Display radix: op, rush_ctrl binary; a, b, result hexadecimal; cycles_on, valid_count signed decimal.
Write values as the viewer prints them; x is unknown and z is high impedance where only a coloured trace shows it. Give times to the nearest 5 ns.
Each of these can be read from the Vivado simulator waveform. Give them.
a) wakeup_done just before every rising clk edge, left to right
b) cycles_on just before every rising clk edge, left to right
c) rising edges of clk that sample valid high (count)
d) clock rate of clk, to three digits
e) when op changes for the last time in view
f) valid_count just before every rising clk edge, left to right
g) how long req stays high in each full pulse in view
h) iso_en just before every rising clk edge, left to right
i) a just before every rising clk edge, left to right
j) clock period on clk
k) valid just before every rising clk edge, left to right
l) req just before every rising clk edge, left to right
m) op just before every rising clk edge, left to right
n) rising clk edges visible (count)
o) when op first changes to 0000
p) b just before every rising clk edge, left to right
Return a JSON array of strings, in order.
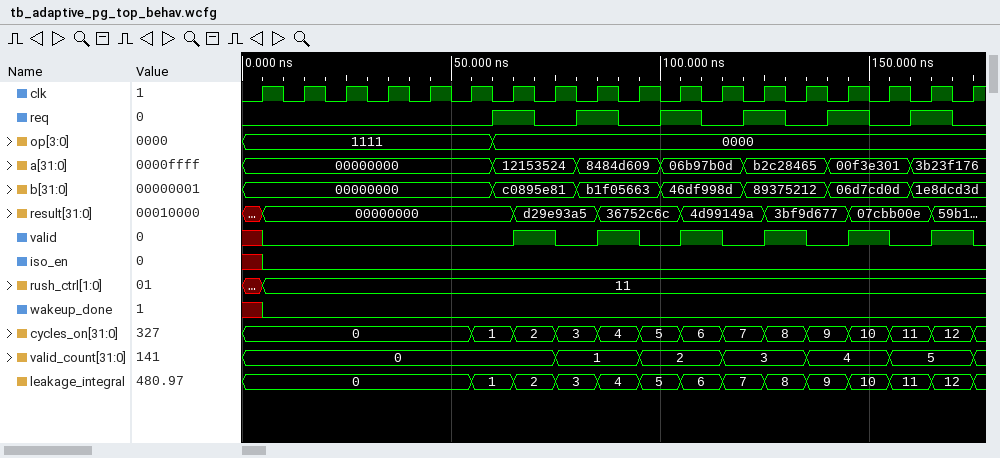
["x 0 0 0 0 0 0 0 0 0 0 0 0 0 0 0 0 0", "0, 0, 0, 0, 0, 0, 1, 2, 3, 4, 5, 6, 7, 8, 9, 10, 11, 12", "6", "100 MHz", "60 ns", "0, 0, 0, 0, 0, 0, 0, 0, 1, 1, 2, 2, 3, 3, 4, 4, 5, 5", "10 ns, 10 ns, 10 ns, 10 ns, 10 ns, 10 ns", "x 0 0 0 0 0 0 0 0 0 0 0 0 0 0 0 0 0", "00000000, 00000000, 00000000, 00000000, 00000000, 00000000, 12153524, 12153524, 8484d609, 8484d609, 06b97b0d, 06b97b0d, b2c28465, b2c28465, 00f3e301, 00f3e301, 3b23f176, 3b23f176", "10 ns", "x 0 0 0 0 0 0 1 0 1 0 1 0 1 0 1 0 1", "0 0 0 0 0 0 1 0 1 0 1 0 1 0 1 0 1 0", "1111, 1111, 1111, 1111, 1111, 1111, 0000, 0000, 0000, 0000, 0000, 0000, 0000, 0000, 0000, 0000, 0000, 0000", "18", "60 ns", "00000000, 00000000, 00000000, 00000000, 00000000, 00000000, c0895e81, c0895e81, b1f05663, b1f05663, 46df998d, 46df998d, 89375212, 89375212, 06d7cd0d, 06d7cd0d, 1e8dcd3d, 1e8dcd3d"]
